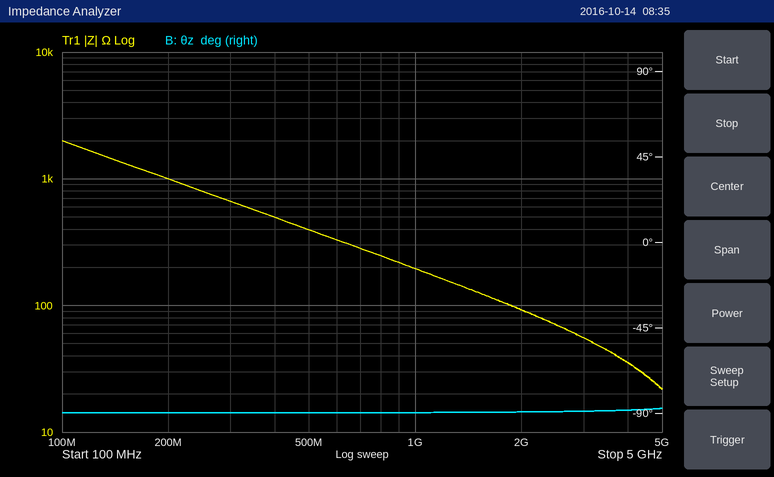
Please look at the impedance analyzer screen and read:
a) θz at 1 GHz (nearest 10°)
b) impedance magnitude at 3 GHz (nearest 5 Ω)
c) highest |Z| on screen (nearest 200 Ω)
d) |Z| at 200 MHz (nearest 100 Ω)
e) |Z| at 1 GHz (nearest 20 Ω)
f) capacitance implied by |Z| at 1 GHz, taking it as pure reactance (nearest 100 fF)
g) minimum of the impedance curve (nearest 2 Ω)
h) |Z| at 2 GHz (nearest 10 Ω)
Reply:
-90°
55 Ω
2.0 kΩ
1.0 kΩ
200 Ω
800 fF
22 Ω
90 Ω
